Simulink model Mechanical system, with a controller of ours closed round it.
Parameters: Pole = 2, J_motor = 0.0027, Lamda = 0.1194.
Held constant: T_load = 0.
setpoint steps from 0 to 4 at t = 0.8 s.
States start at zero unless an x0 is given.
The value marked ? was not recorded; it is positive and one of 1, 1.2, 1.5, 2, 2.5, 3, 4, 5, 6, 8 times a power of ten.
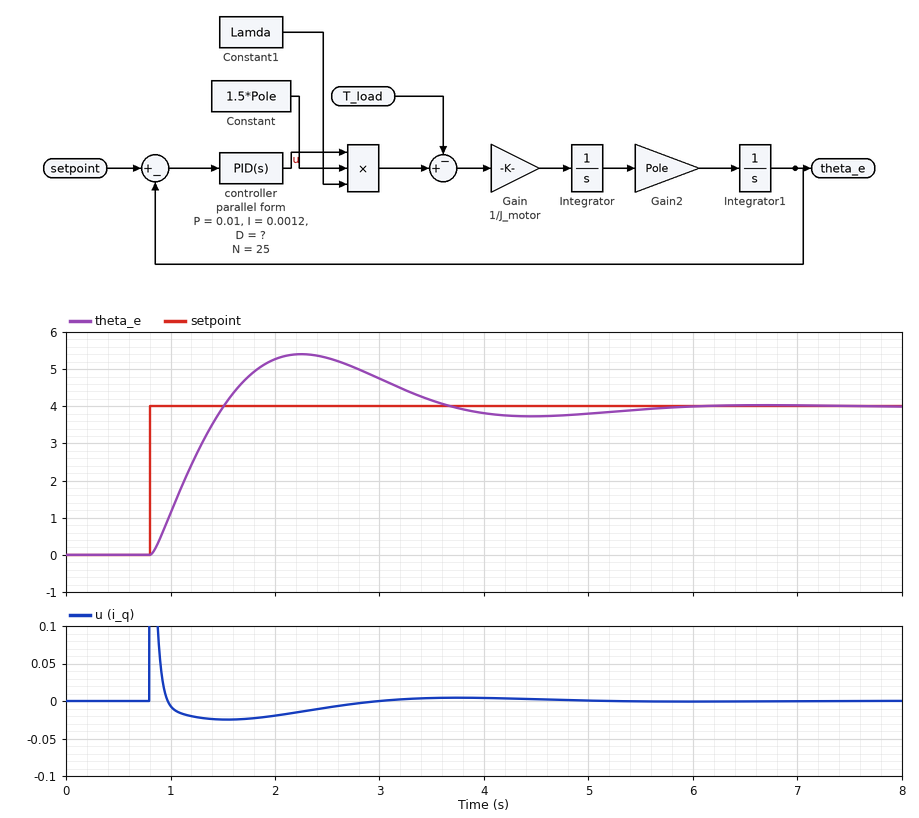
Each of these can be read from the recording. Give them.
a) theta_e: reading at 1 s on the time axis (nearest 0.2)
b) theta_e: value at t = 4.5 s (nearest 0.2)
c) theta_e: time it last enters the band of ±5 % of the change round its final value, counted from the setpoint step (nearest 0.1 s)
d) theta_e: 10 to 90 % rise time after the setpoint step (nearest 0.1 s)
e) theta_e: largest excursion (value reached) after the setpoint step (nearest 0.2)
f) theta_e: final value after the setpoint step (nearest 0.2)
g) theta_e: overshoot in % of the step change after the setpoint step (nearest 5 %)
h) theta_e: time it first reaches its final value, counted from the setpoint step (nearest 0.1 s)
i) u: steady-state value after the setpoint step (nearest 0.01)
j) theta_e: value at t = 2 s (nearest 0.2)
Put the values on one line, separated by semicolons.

1.2; 3.8; 4.2 s; 0.5 s; 5.4; 4.0; 35 %; 0.7 s; 0.00; 5.2
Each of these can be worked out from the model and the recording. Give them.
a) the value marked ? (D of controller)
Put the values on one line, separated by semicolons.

0.006
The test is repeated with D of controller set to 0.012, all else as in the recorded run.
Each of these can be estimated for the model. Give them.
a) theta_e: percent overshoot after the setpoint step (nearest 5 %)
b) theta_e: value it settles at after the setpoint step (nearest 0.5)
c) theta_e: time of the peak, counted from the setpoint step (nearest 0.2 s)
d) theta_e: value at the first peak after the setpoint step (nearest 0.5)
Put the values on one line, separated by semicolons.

15 %; 4.0; 1.2 s; 4.5
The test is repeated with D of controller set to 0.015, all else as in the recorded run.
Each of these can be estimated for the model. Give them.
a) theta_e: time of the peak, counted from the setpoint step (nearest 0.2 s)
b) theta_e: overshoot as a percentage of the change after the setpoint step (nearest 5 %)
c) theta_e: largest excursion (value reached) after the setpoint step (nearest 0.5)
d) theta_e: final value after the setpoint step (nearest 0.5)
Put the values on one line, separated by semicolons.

1.0 s; 10 %; 4.5; 4.0
